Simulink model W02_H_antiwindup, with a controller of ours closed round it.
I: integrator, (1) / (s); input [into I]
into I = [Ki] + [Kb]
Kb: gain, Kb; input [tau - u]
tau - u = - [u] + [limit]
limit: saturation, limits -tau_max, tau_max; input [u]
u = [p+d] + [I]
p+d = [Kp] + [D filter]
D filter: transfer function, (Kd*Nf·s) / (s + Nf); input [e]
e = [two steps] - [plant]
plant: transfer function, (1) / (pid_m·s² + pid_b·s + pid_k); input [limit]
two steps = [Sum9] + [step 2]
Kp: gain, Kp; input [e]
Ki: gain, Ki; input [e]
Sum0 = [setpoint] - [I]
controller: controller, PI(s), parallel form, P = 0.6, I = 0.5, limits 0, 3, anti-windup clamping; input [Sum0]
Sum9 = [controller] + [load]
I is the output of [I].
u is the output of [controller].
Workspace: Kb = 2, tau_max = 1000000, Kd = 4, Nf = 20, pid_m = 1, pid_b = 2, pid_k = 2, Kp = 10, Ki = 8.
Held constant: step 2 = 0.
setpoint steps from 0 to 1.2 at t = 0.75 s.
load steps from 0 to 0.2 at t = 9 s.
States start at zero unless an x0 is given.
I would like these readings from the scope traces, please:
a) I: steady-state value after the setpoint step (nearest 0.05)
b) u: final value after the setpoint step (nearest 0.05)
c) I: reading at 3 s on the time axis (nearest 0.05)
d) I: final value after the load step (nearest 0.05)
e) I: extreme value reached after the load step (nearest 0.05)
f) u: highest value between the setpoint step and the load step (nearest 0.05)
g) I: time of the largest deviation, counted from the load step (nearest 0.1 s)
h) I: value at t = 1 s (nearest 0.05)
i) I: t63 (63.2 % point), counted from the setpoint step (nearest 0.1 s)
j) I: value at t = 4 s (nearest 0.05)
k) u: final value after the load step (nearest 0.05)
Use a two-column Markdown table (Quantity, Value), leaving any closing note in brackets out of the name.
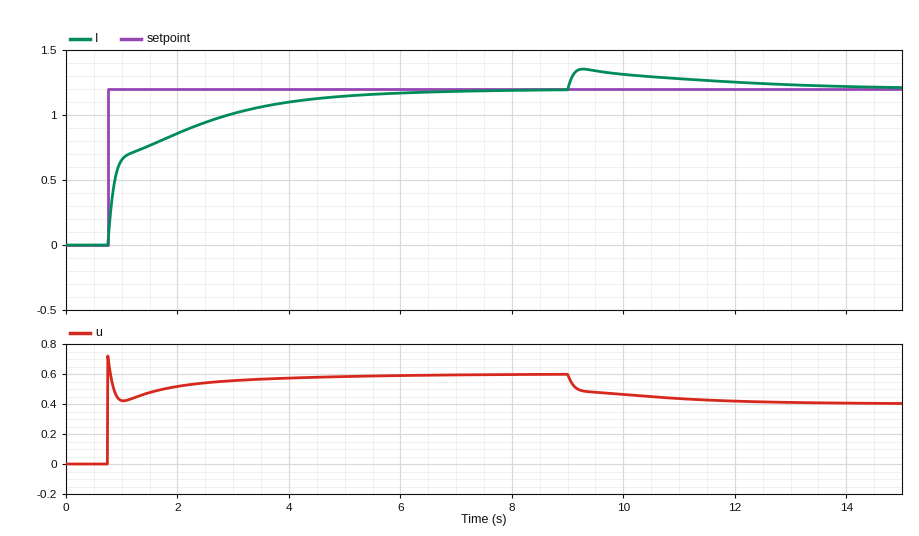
| Quantity | Value |
|---|---|
| I: steady-state value after the setpoint step | 1.20 |
| u: final value after the setpoint step | 0.60 |
| I: reading at 3 s on the time axis | 1.00 |
| I: final value after the load step | 1.20 |
| I: extreme value reached after the load step | 1.35 |
| u: highest value between the setpoint step and the load step | 0.70 |
| I: time of the largest deviation, counted from the load step | 0.3 s |
| I: value at t = 1 s | 0.65 |
| I: t63 (63.2 % point), counted from the setpoint step | 0.7 s |
| I: value at t = 4 s | 1.10 |
| u: final value after the load step | 0.40 |
